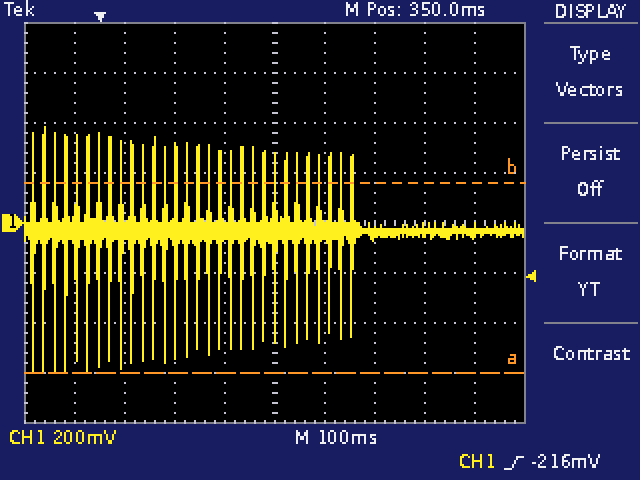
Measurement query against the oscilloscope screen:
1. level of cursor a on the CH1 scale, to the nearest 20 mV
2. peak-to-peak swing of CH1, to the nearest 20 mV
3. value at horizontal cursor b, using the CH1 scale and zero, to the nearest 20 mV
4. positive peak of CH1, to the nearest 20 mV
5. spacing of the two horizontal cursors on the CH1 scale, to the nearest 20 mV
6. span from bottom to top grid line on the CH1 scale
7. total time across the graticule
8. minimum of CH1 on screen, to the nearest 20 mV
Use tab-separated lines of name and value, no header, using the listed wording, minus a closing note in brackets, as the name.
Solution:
level of cursor a on the CH1 scale, to the nearest 20 mV	-600 mV
peak-to-peak swing of CH1, to the nearest 20 mV	980 mV
value at horizontal cursor b, using the CH1 scale and zero, to the nearest 20 mV	160 mV
positive peak of CH1, to the nearest 20 mV	380 mV
spacing of the two horizontal cursors on the CH1 scale, to the nearest 20 mV	760 mV
span from bottom to top grid line on the CH1 scale	1.6 V
total time across the graticule	1 s
minimum of CH1 on screen, to the nearest 20 mV	-600 mV
